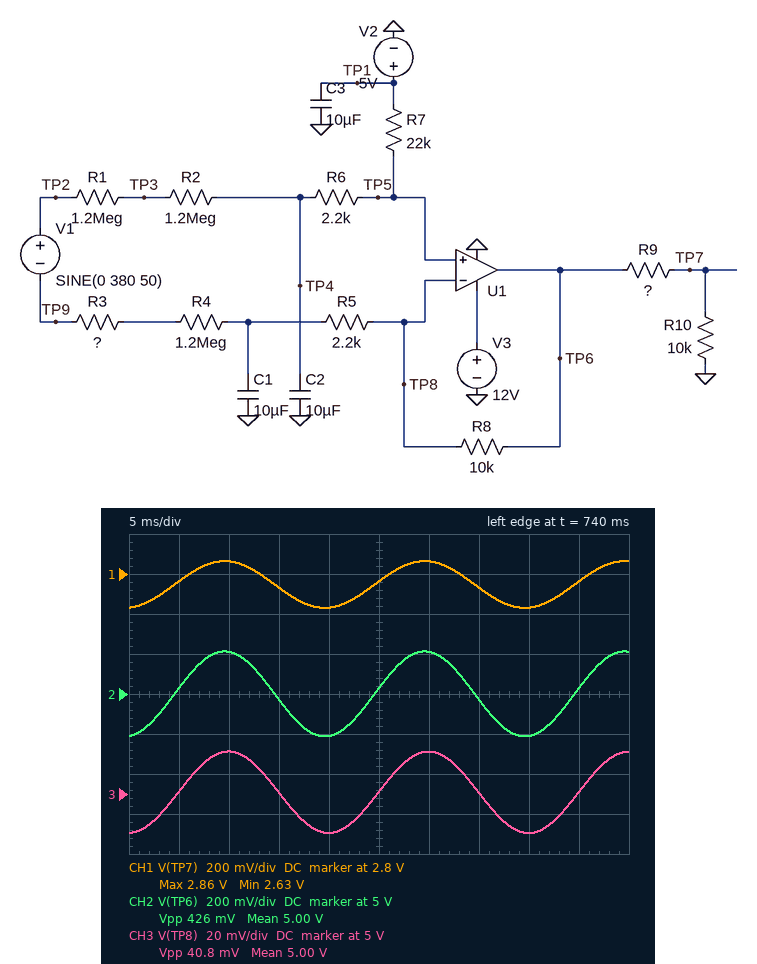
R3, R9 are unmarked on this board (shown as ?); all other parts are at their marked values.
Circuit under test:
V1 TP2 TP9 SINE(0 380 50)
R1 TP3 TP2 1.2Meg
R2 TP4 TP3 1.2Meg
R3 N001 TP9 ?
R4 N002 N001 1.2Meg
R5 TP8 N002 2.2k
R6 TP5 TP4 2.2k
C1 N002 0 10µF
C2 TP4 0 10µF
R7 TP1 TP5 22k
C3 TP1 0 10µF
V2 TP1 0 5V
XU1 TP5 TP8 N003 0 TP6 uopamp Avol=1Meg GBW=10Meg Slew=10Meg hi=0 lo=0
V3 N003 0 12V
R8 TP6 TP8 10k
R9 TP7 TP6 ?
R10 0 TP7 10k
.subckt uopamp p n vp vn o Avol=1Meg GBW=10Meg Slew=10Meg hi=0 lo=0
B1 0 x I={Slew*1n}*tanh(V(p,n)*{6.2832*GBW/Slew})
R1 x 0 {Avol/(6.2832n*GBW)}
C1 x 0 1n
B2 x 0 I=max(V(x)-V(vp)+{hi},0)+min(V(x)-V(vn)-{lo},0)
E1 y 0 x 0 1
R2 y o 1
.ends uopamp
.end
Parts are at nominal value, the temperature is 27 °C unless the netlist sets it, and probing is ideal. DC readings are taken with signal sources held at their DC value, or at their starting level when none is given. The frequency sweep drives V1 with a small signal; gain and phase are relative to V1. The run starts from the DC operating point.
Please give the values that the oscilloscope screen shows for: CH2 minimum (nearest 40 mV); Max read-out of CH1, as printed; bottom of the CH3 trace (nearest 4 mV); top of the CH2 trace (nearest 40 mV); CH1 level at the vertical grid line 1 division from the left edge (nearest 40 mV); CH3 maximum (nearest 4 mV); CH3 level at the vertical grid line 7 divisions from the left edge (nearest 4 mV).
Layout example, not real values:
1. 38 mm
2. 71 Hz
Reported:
1. 4.80 V
2. 2.86 V
3. 4.980 V
4. 5.20 V
5. 2.76 V
6. 5.020 V
7. 5.000 V
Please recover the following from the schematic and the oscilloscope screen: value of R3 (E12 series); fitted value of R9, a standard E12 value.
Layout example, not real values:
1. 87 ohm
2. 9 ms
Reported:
1. 1.8 MΩ
2. 8.2 kΩ
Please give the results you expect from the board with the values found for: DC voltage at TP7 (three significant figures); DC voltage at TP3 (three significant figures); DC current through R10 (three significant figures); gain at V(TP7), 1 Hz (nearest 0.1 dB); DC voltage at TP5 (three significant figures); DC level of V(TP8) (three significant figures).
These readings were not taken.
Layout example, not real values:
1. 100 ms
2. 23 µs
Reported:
1. 2.75 V
2. 5.00 V
3. 275 µA
4. -52.0 dB
5. 5.00 V
6. 5.00 V
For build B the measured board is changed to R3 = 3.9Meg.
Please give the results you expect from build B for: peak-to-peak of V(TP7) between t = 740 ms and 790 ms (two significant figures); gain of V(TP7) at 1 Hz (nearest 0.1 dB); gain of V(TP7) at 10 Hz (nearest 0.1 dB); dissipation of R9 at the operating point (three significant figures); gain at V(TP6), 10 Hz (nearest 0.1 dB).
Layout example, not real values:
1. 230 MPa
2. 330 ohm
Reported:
1. 170 mV
2. -54.9 dB
3. -60.8 dB
4. 619 µW
5. -55.6 dB
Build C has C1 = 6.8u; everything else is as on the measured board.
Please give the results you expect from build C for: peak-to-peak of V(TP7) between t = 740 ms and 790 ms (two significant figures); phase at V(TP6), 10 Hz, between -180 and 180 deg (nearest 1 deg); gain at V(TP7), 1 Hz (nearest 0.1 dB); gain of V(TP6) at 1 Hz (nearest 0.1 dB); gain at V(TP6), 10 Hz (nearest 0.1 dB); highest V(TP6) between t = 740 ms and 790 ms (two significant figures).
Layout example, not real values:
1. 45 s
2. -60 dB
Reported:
1. 280 mV
2. -46 deg
3. -52.7 dB
4. -47.5 dB
5. -52.5 dB
6. 5.3 V
